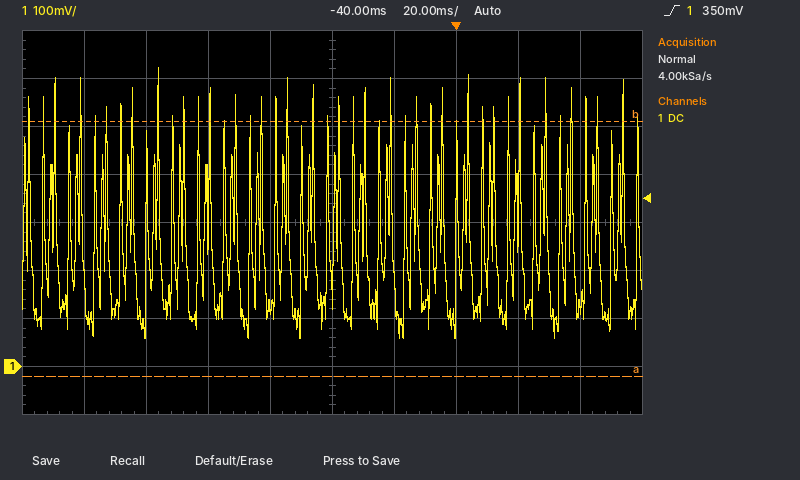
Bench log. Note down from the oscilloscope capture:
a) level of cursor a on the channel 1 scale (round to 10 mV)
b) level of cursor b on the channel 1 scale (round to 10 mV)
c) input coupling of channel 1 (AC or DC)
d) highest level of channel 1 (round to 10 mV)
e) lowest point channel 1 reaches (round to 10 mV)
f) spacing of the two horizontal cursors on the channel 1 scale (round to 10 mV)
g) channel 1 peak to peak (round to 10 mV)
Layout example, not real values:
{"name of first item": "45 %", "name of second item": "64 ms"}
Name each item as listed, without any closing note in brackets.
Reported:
{"level of cursor a on the channel 1 scale": "-20 mV", "level of cursor b on the channel 1 scale": "510 mV", "input coupling of channel 1": "DC", "highest level of channel 1": "620 mV", "lowest point channel 1 reaches": "60 mV", "spacing of the two horizontal cursors on the channel 1 scale": "530 mV", "channel 1 peak to peak": "560 mV"}
